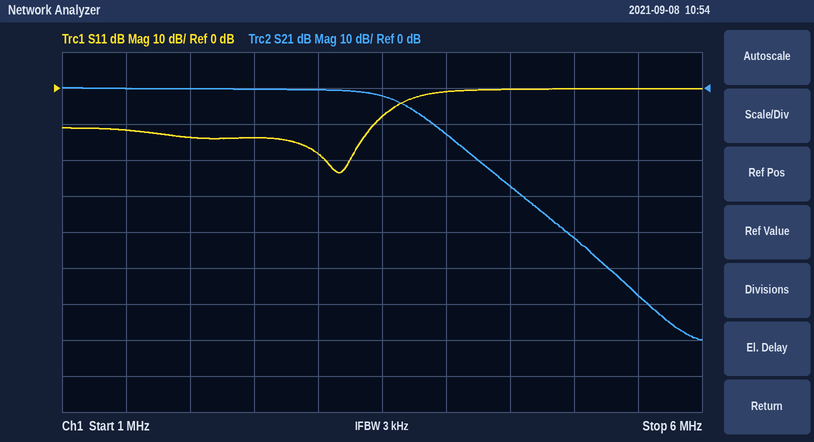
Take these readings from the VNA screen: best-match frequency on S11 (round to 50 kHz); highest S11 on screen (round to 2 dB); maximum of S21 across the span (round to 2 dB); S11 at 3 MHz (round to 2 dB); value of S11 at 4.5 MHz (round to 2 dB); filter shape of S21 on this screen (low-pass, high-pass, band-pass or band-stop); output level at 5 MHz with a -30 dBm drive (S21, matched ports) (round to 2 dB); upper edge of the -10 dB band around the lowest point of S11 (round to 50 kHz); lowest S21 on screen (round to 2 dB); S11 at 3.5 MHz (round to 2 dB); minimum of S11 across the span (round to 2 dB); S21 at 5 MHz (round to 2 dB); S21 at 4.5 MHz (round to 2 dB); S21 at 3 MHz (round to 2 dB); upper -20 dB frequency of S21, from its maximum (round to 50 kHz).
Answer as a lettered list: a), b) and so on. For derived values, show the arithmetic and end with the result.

a) 3.15 MHz
b) 0 dB
c) 0 dB
d) -18 dB
e) 0 dB
f) low-pass
g) -30 dBm + (-42 dB) = -72 dBm
h) 3.45 MHz
i) -70 dB
j) -8 dB
k) -24 dB
l) -42 dB
m) -28 dB
n) 0 dB
o) 4.25 MHz
